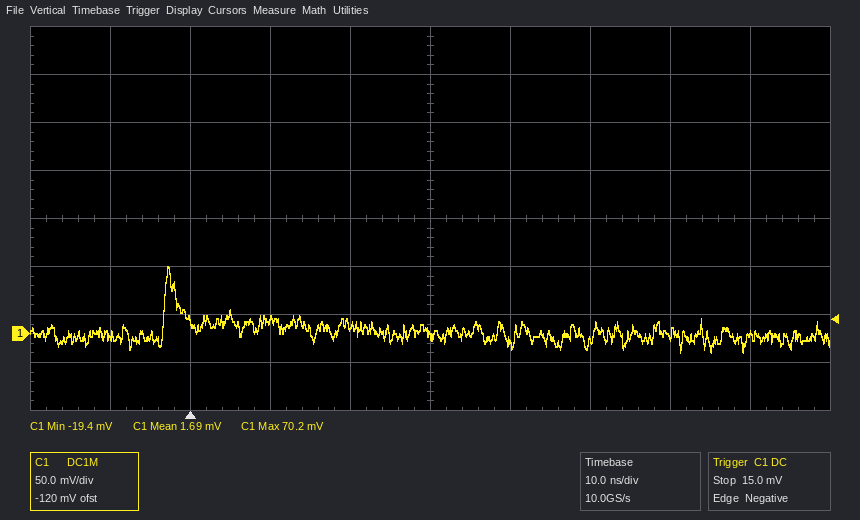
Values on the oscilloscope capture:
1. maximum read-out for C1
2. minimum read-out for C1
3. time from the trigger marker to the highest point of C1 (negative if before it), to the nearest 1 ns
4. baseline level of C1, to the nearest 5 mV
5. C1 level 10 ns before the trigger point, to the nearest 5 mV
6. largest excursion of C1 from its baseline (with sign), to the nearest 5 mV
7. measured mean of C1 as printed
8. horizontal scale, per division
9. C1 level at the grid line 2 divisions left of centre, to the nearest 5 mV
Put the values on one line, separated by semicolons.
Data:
70.2 mV; -19.4 mV; -3 ns; 0 mV; 0 mV; +70 mV; 1.69 mV; 10 ns; 15 mV
